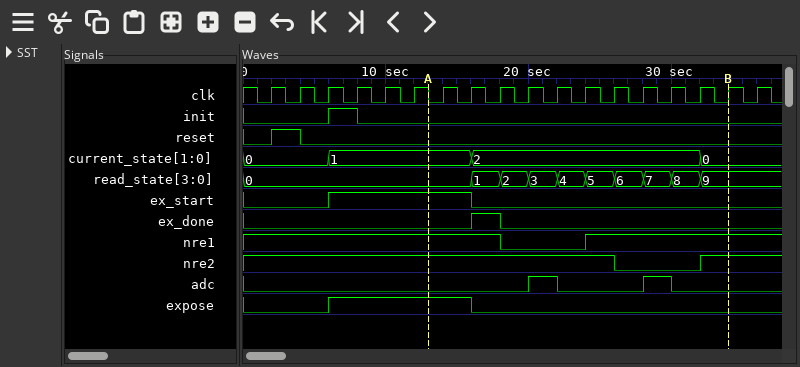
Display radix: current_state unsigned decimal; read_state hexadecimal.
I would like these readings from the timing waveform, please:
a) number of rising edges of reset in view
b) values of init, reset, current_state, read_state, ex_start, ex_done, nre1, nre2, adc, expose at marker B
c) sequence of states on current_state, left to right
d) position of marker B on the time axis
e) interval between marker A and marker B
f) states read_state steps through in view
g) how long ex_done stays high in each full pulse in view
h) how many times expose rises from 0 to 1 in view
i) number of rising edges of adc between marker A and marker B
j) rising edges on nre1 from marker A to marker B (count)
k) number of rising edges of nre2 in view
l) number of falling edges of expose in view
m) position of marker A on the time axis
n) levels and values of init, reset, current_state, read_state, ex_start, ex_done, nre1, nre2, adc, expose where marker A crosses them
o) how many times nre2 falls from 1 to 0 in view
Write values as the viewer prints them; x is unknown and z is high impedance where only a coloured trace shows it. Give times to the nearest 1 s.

1
init=0, reset=0, current_state=0, read_state=9, ex_start=0, ex_done=0, nre1=1, nre2=1, adc=0, expose=0
0, 1, 2, 0
34 s
21 s
0, 1, 2, 3, 4, 5, 6, 7, 8, 9
2 s
1
2
1
1
1
13 s
init=0, reset=0, current_state=1, read_state=0, ex_start=1, ex_done=0, nre1=1, nre2=1, adc=0, expose=1
1
